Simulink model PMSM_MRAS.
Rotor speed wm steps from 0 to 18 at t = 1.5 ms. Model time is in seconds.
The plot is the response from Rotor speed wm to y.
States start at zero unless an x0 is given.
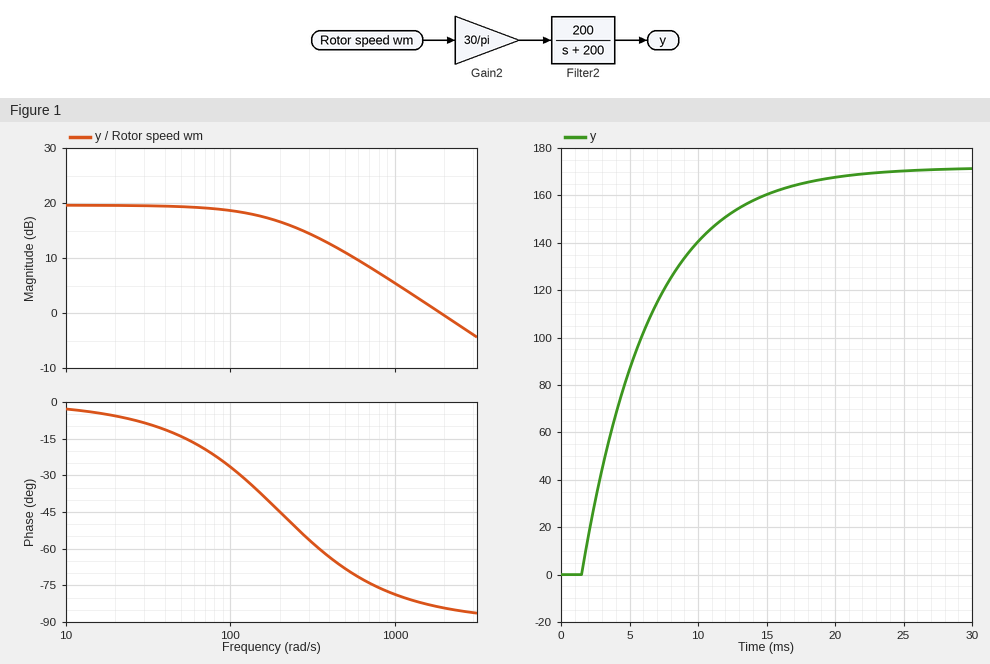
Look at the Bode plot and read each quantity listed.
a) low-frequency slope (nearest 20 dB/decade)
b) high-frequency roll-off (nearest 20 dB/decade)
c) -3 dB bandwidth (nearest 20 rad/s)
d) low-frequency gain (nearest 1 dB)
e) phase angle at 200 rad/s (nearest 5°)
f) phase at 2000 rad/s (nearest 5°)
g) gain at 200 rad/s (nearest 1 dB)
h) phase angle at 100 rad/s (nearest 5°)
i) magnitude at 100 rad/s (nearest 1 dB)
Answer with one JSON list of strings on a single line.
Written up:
["0 dB/decade", "-20 dB/decade", "200 rad/s", "20 dB", "-45°", "-85°", "17 dB", "-25°", "19 dB"]
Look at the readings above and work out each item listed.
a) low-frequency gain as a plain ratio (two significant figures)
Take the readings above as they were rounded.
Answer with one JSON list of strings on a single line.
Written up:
["10"]
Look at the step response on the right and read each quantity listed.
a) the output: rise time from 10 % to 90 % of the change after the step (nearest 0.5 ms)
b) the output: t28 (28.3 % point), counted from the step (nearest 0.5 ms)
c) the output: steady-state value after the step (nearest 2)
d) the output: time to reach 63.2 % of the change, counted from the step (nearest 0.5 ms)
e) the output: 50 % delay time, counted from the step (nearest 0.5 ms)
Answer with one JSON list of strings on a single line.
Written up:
["11.0 ms", "1.5 ms", "172", "5.0 ms", "3.5 ms"]
